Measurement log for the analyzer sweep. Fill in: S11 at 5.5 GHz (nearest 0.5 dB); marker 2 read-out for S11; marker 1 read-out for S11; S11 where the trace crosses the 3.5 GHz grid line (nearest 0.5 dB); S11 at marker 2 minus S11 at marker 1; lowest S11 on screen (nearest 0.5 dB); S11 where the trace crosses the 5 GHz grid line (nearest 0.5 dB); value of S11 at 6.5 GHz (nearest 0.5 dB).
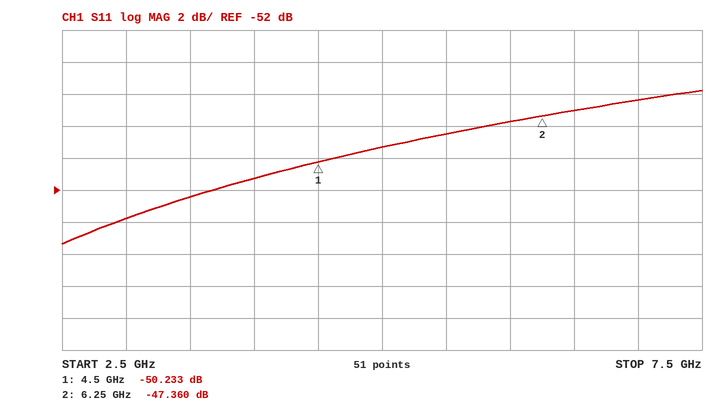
-48.5 dB
-47.360 dB
-50.233 dB
-52.5 dB
2.873 dB
-55.5 dB
-49.5 dB
-47.0 dB
